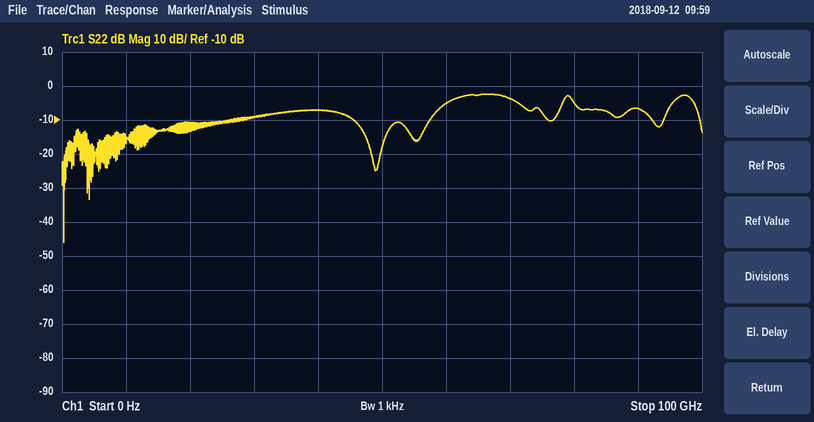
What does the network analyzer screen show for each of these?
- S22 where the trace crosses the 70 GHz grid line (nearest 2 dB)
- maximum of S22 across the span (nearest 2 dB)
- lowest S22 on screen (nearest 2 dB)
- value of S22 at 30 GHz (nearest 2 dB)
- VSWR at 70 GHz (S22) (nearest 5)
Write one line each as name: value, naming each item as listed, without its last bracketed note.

S22 where the trace crosses the 70 GHz grid line: -4 dB
maximum of S22 across the span: -2 dB
lowest S22 on screen: -46 dB
value of S22 at 30 GHz: -10 dB
VSWR at 70 GHz (S22): 5
